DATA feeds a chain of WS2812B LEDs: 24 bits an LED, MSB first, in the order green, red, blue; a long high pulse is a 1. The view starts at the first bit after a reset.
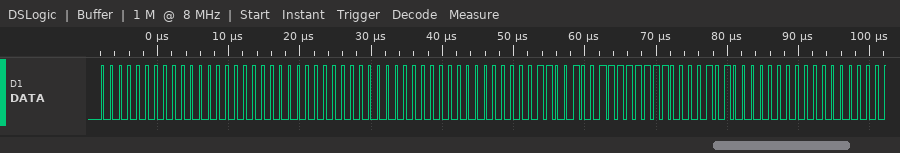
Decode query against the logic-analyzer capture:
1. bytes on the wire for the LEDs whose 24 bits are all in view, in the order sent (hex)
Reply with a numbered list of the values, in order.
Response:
1. 00 00 00 00 00 00 64 FF 0A
